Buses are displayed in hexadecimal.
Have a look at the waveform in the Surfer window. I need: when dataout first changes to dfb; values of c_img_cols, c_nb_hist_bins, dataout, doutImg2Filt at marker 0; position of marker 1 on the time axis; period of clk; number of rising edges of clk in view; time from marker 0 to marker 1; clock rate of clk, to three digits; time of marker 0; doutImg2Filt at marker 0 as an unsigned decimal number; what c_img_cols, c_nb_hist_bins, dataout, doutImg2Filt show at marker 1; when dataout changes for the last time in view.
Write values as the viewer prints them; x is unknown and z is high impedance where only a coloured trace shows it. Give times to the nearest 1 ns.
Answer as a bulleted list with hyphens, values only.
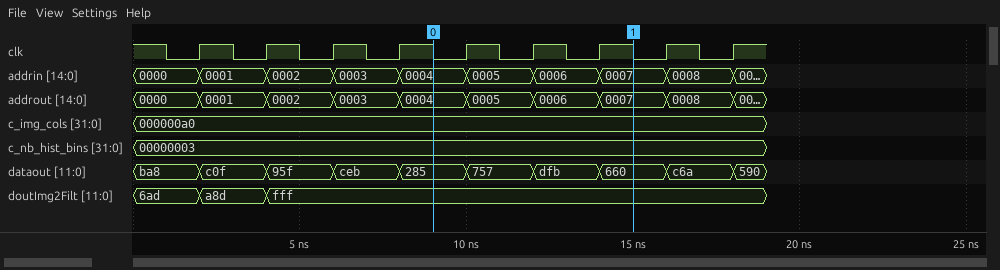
- 12 ns
- c_img_cols=000000a0, c_nb_hist_bins=00000003, dataout=285, doutImg2Filt=fff
- 15 ns
- 2 ns
- 9
- 6 ns
- 500 MHz
- 9 ns
- 4095
- c_img_cols=000000a0, c_nb_hist_bins=00000003, dataout=660, doutImg2Filt=fff
- 18 ns
